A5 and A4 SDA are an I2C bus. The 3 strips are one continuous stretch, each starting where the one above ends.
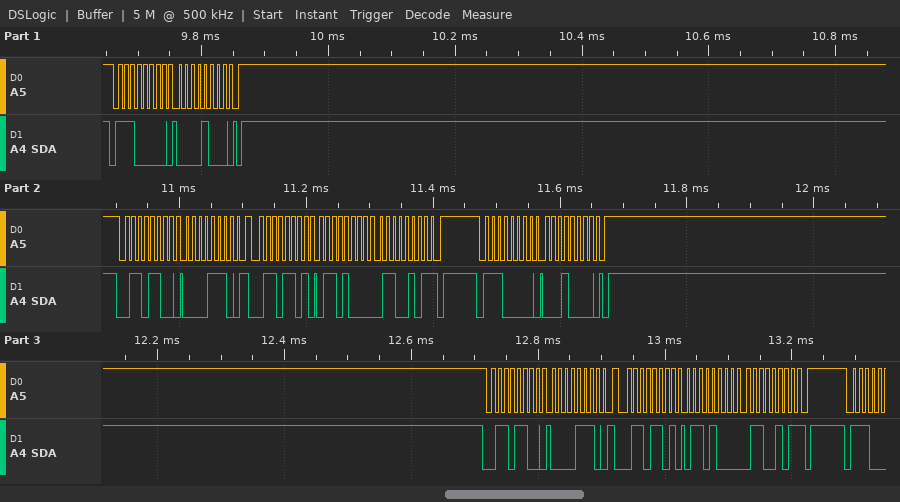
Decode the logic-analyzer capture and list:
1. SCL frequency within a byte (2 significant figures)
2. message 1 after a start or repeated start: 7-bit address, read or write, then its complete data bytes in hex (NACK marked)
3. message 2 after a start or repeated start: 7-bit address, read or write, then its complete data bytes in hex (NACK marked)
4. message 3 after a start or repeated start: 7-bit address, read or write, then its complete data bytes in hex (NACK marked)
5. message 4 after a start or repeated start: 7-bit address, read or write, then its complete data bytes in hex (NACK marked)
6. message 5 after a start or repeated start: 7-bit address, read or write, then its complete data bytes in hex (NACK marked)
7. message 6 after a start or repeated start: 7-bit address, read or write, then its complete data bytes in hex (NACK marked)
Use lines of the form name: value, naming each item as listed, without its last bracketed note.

SCL frequency within a byte: 100 kHz
message 1 after a start or repeated start: 7-bit address, read or write, then its complete data bytes in hex: 0x70 write: 08
message 2 after a start or repeated start: 7-bit address, read or write, then its complete data bytes in hex: 0x36 write: 0E
message 3 after a start or repeated start: 7-bit address, read or write, then its complete data bytes in hex: 0x36 read: 68 65 NACK
message 4 after a start or repeated start: 7-bit address, read or write, then its complete data bytes in hex: 0x70 write: 10
message 5 after a start or repeated start: 7-bit address, read or write, then its complete data bytes in hex: 0x36 write: 0E
message 6 after a start or repeated start: 7-bit address, read or write, then its complete data bytes in hex: 0x36 read: 68 65 NACK
